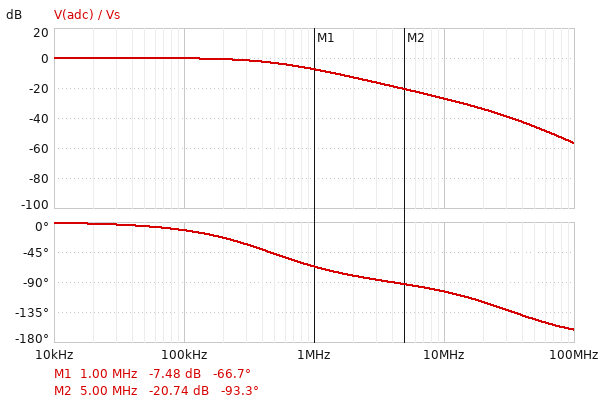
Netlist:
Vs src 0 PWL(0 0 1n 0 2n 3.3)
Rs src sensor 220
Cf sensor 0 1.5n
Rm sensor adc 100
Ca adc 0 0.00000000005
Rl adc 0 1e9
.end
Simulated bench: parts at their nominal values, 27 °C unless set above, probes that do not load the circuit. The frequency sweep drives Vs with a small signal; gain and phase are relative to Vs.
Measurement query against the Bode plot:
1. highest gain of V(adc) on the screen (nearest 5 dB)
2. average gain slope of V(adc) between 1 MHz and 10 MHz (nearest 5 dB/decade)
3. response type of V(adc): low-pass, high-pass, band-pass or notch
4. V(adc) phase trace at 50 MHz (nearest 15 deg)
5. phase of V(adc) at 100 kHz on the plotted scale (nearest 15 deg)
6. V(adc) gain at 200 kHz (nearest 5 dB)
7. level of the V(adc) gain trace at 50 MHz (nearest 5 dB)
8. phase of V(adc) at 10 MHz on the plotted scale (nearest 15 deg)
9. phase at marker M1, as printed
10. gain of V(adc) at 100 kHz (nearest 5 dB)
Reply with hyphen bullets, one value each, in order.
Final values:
- 0 dB
- -20 dB/decade
- low-pass
- -150 deg
- -15 deg
- 0 dB
- -45 dB
- -105 deg
- -66.7 deg
- 0 dB
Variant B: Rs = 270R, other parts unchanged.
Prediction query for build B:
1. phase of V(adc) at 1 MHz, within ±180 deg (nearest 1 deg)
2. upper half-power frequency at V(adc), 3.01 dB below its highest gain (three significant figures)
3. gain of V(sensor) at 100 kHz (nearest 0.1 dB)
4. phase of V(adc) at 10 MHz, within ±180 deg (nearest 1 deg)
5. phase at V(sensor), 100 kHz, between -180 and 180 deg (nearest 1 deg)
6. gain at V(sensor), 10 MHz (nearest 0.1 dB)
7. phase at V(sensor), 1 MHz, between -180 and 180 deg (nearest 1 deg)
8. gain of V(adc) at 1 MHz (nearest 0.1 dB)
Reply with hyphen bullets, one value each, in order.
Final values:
- -71 deg
- 380 kHz
- -0.3 dB
- -105 deg
- -15 deg
- -28.4 dB
- -69 deg
- -9.0 dB
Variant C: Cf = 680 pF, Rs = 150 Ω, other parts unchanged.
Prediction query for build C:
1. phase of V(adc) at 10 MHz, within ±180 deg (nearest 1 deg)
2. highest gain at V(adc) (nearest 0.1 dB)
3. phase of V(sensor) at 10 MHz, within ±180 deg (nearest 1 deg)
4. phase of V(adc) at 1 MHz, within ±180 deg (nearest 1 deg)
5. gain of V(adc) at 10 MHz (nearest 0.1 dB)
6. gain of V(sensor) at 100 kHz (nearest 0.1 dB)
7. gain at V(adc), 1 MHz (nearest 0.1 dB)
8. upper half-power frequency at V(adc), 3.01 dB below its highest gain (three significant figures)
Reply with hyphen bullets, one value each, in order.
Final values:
- -98 deg
- 0 dB
- -81 deg
- -36 deg
- -17.2 dB
- 0 dB
- -1.7 dB
- 1.45 MHz
